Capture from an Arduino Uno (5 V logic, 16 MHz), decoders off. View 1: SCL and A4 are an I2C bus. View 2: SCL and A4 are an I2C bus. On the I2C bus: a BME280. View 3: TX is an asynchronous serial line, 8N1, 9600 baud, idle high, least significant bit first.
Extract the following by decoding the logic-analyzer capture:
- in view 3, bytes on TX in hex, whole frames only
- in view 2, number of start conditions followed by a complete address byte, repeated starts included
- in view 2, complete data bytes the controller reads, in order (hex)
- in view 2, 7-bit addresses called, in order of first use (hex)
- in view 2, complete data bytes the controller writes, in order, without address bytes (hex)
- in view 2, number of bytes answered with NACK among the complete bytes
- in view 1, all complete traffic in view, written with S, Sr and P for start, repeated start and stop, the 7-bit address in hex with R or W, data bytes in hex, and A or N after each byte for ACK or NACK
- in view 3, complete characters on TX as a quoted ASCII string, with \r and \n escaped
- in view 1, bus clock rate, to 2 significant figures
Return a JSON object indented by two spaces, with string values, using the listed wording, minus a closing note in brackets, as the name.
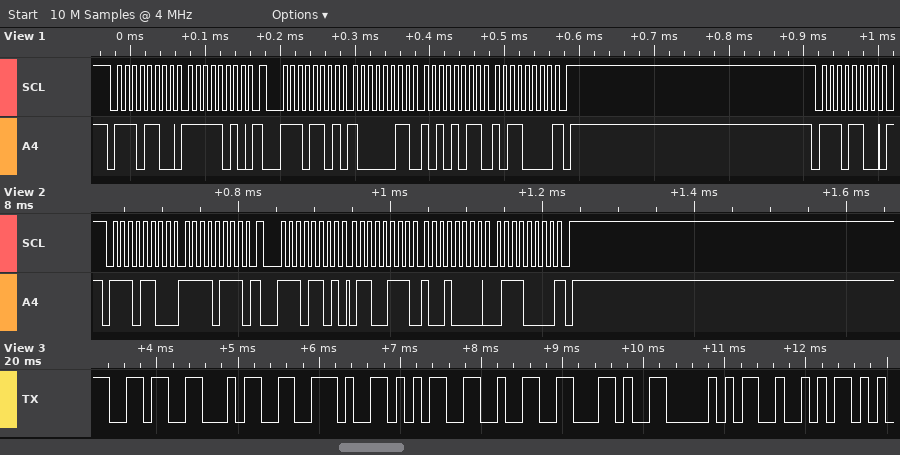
{
  "in view 3, bytes on TX in hex, whole frames only": "36 34 2E 35 32 2C 50 52",
  "in view 2, number of start conditions followed by a complete address byte, repeated starts included": "2",
  "in view 2, complete data bytes the controller reads, in order": "67 90 70",
  "in view 2, 7-bit addresses called, in order of first use": "0x76",
  "in view 2, complete data bytes the controller writes, in order, without address bytes": "F7",
  "in view 2, number of bytes answered with NACK among the complete bytes": "1",
  "in view 1, all complete traffic in view, written with S, Sr and P for start, repeated start and stop, the 7-bit address in hex with R or W, data bytes in hex, and A or N after each byte for ACK or NACK": "S 76W A FA A Sr 76R A 83 A AB A B0 N P S 76W A",
  "in view 3, complete characters on TX as a quoted ASCII string, with \\r and \\n escaped": "\"64.52,PR\"",
  "in view 1, bus clock rate, to 2 significant figures": "100 kHz"
}
